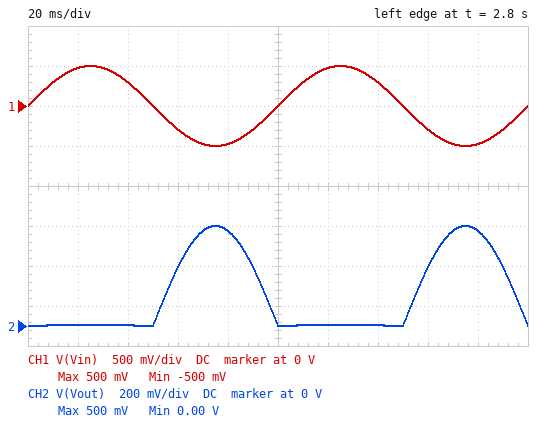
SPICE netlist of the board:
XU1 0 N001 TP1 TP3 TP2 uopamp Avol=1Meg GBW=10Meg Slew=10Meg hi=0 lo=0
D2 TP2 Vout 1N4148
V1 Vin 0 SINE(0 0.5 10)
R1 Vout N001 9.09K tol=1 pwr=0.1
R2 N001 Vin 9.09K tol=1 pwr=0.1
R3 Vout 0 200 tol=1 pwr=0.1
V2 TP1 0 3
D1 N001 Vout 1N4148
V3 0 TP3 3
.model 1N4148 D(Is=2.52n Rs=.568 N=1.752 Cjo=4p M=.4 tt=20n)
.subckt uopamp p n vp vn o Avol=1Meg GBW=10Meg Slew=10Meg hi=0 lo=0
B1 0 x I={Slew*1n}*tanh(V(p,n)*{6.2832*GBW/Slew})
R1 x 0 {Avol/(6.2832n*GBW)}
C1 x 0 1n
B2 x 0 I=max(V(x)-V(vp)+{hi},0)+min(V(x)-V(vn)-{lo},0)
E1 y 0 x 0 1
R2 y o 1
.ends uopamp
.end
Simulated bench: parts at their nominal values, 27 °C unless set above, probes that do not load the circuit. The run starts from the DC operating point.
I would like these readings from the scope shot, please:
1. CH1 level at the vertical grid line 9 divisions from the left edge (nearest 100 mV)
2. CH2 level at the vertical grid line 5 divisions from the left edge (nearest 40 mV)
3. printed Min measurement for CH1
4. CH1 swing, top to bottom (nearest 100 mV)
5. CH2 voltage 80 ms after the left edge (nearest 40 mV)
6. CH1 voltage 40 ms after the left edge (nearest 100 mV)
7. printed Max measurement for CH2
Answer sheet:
-500 mV
0 V
-500 mV
1.0 V
480 mV
300 mV
500 mV
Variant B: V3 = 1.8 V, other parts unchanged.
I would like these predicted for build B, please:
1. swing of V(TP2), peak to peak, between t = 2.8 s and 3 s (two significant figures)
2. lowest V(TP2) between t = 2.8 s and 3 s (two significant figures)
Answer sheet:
2.9 V
-1.8 V
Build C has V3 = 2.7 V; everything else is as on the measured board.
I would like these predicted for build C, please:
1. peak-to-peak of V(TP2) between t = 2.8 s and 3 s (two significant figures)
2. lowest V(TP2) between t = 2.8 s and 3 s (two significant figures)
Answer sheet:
3.8 V
-2.7 V
